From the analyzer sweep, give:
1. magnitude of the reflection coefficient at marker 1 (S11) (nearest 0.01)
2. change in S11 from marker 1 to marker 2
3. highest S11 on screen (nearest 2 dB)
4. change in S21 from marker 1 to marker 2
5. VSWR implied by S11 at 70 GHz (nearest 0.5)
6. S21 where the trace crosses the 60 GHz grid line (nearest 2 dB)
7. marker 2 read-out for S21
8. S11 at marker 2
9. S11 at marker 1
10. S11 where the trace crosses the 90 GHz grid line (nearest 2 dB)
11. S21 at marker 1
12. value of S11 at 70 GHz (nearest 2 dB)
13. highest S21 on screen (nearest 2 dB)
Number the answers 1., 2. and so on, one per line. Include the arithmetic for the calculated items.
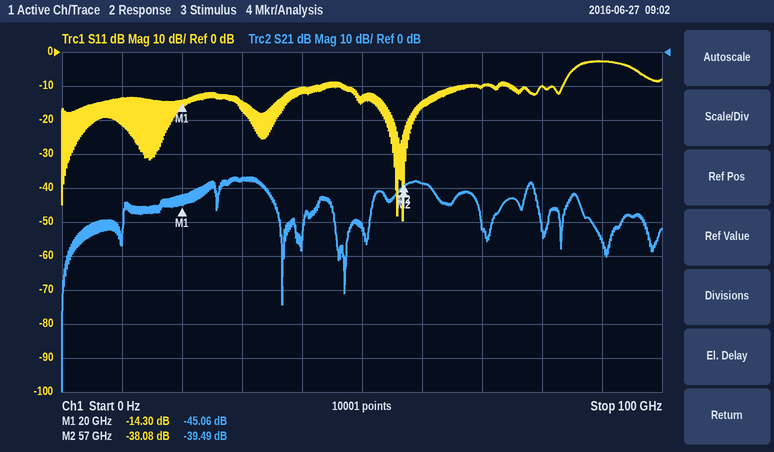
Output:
1. 10^(-14.3/20) ≈ 0.19
2. -38.08 − (-14.3) = -23.78 dB
3. -2 dB
4. -39.49 − (-45.06) = 5.57 dB
5. |Γ| = 10^(-10/20) = 0.3162; VSWR = (1 + 0.3162)/(1 − 0.3162) ≈ 1.92, so 2.0 to the nearest 0.5
6. -38 dB
7. -39.49 dB
8. -38.08 dB
9. -14.30 dB
10. -2 dB
11. -45.06 dB
12. -10 dB
13. -36 dB
